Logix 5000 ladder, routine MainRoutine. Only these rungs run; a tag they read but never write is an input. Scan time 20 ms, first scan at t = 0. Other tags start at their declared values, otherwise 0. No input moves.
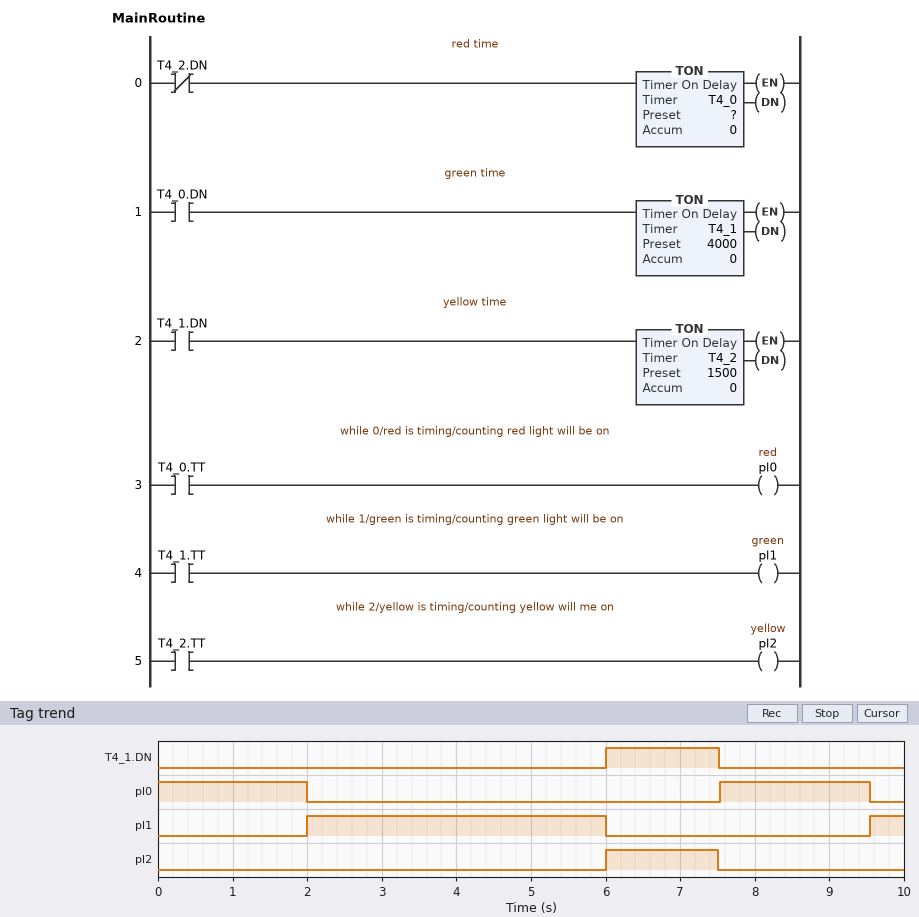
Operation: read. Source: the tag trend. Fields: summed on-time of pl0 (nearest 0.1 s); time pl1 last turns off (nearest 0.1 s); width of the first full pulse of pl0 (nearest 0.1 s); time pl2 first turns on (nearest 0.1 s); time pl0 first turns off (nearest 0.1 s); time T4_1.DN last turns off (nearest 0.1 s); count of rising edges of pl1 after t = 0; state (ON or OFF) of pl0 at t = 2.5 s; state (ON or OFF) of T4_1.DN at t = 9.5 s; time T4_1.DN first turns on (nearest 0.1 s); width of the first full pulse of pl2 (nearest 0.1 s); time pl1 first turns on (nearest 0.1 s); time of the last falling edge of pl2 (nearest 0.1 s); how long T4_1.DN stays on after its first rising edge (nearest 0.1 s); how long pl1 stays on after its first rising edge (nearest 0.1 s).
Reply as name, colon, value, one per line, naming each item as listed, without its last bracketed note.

summed on-time of pl0: 4.0 s
time pl1 last turns off: 6.0 s
width of the first full pulse of pl0: 2.0 s
time pl2 first turns on: 6.0 s
time pl0 first turns off: 2.0 s
time T4_1.DN last turns off: 7.5 s
count of rising edges of pl1 after t = 0: 2
state (ON or OFF) of pl0 at t = 2.5 s: OFF
state (ON or OFF) of T4_1.DN at t = 9.5 s: OFF
time T4_1.DN first turns on: 6.0 s
width of the first full pulse of pl2: 1.5 s
time pl1 first turns on: 2.0 s
time of the last falling edge of pl2: 7.5 s
how long T4_1.DN stays on after its first rising edge: 1.5 s
how long pl1 stays on after its first rising edge: 4.0 s
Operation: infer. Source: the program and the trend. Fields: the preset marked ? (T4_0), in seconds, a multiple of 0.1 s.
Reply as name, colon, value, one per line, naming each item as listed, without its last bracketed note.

the preset marked ? (T4_0), in seconds, a multiple of 0.1 s: 2.0 s
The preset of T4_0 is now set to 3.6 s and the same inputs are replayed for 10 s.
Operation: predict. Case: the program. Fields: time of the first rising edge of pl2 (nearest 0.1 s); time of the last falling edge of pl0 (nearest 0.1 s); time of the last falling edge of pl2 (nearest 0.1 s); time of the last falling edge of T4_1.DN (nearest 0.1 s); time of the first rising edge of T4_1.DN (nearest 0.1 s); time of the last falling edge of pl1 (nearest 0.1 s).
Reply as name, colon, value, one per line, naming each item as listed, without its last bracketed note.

time of the first rising edge of pl2: 7.6 s
time of the last falling edge of pl0: 3.6 s
time of the last falling edge of pl2: 9.1 s
time of the last falling edge of T4_1.DN: 9.1 s
time of the first rising edge of T4_1.DN: 7.6 s
time of the last falling edge of pl1: 7.6 s
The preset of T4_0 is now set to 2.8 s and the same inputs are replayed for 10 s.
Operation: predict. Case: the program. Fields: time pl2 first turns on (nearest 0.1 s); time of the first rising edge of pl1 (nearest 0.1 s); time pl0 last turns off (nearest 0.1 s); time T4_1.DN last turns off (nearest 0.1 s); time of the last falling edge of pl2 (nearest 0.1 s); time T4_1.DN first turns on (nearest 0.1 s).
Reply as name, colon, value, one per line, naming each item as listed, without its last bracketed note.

time pl2 first turns on: 6.8 s
time of the first rising edge of pl1: 2.8 s
time pl0 last turns off: 2.8 s
time T4_1.DN last turns off: 8.3 s
time of the last falling edge of pl2: 8.3 s
time T4_1.DN first turns on: 6.8 s
